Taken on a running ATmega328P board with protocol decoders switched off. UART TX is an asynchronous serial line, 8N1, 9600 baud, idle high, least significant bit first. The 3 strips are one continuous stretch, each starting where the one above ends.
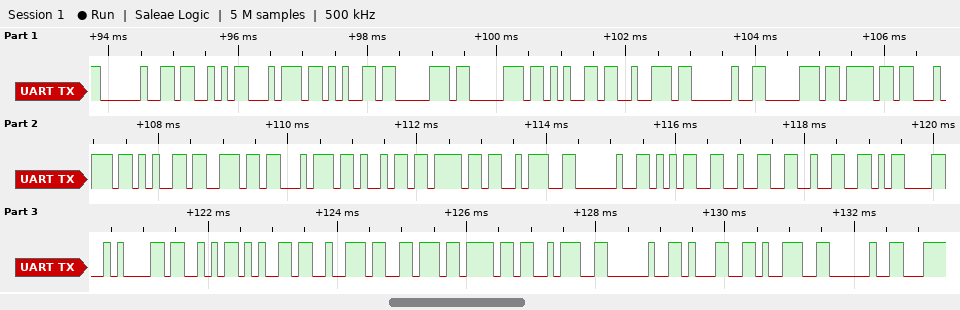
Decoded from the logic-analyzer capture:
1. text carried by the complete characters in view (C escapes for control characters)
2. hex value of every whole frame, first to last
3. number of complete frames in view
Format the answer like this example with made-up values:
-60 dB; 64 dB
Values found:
" Stepper potentio: 522\r\nServo: 19 "; 20 53 74 65 70 70 65 72 20 70 6F 74 65 6E 74 69 6F 3A 20 35 32 32 0D 0A 53 65 72 76 6F 3A 20 31 39 20; 34
